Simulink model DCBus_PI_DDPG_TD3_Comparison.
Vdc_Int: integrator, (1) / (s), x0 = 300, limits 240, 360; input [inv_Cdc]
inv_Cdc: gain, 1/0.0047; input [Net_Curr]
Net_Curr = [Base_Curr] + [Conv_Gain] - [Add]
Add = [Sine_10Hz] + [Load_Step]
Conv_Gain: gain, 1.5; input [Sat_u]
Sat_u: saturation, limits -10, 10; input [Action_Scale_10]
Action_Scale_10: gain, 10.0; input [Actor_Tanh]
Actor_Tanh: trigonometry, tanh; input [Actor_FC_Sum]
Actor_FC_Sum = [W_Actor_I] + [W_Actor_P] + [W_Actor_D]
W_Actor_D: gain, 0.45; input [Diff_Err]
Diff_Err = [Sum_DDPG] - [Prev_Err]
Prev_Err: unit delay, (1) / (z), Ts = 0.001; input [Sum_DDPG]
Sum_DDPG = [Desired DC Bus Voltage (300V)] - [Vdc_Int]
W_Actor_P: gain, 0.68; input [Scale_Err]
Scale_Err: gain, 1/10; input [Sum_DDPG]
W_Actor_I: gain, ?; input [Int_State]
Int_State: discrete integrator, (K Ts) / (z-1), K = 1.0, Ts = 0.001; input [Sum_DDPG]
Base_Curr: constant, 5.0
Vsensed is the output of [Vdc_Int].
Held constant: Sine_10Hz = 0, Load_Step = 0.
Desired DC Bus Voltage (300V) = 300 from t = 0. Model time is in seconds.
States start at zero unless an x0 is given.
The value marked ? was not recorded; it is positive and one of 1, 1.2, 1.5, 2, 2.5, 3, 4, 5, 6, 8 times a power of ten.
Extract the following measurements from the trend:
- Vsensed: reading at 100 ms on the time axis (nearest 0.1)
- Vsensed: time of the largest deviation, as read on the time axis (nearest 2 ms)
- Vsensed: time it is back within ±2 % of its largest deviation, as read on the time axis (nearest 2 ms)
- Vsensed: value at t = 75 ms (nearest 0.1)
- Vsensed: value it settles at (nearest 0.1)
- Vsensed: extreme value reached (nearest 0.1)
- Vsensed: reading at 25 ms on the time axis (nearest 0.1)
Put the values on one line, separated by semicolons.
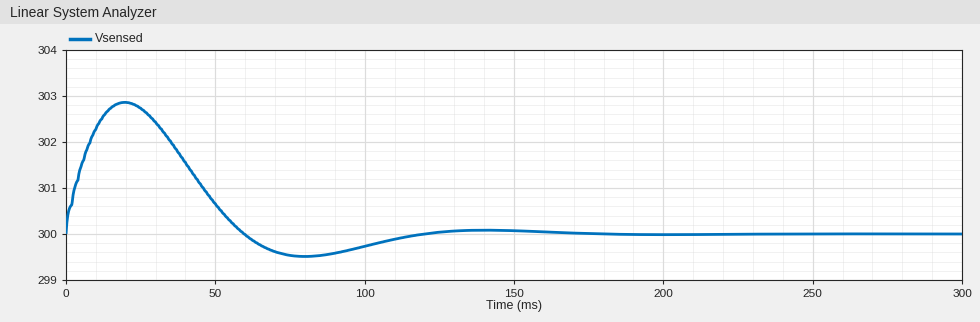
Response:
299.7; 20 ms; 156 ms; 299.5; 300.0; 302.9; 302.7
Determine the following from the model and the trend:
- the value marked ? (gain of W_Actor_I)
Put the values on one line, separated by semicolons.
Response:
4
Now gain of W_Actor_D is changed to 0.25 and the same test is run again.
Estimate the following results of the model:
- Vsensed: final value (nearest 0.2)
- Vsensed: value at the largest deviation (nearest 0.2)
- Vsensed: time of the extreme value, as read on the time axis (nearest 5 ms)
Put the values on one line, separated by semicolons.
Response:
300.0; 303.2; 15 ms
